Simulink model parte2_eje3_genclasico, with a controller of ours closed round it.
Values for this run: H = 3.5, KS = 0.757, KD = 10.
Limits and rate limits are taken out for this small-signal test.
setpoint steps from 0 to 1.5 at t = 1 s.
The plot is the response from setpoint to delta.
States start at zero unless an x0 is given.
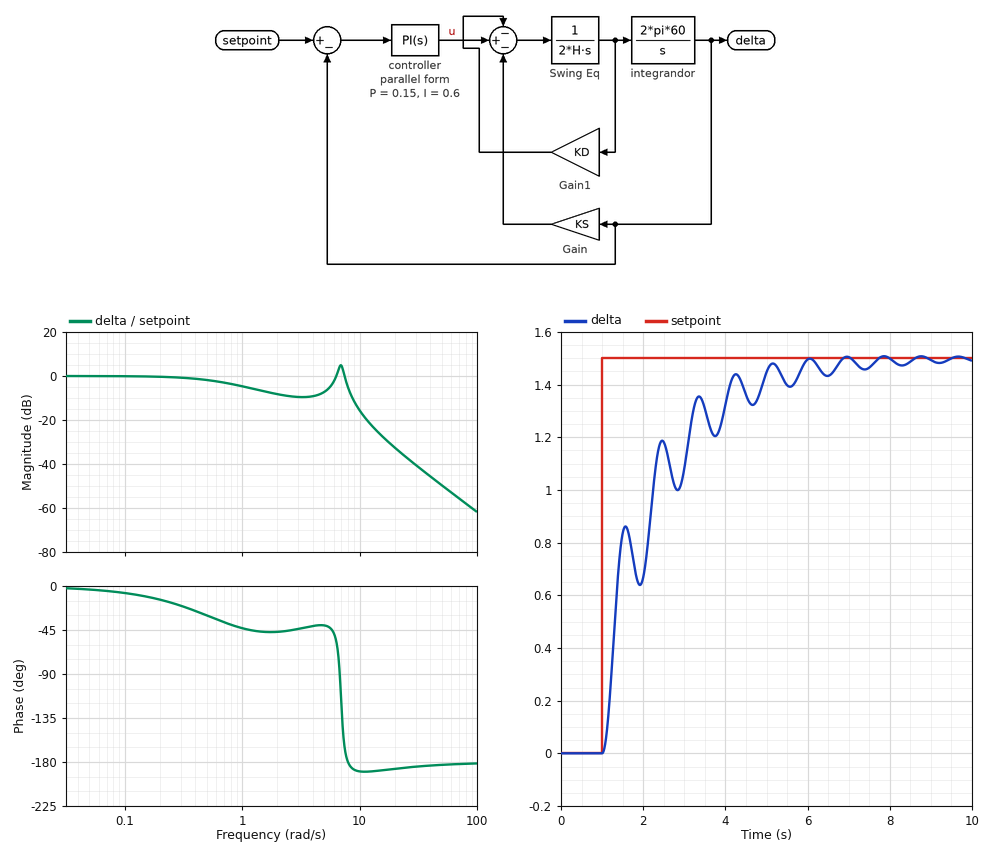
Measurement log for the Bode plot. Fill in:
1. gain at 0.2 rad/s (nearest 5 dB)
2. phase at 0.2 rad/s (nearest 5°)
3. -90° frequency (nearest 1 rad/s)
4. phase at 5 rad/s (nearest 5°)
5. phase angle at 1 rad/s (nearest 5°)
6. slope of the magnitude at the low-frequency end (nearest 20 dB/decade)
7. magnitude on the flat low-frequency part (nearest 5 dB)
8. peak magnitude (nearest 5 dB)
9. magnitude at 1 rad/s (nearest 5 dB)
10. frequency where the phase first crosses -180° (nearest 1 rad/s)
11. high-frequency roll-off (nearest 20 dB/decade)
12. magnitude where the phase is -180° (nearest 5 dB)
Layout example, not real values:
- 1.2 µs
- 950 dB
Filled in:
- 0 dB
- -15°
- 7 rad/s
- -40°
- -45°
- 0 dB/decade
- 0 dB
- 5 dB
- -5 dB
- 8 rad/s
- -40 dB/decade
- -5 dB
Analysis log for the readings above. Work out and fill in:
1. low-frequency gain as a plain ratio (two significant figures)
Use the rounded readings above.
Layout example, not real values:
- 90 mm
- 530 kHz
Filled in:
- 1.0
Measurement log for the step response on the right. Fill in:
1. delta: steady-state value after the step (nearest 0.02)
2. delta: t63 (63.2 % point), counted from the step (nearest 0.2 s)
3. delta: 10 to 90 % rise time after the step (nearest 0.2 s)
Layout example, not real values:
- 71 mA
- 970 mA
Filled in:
- 1.50
- 1.2 s
- 2.2 s
